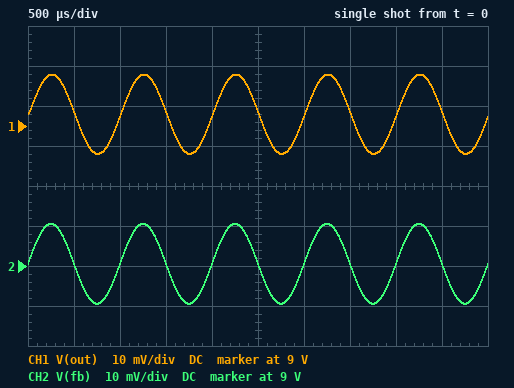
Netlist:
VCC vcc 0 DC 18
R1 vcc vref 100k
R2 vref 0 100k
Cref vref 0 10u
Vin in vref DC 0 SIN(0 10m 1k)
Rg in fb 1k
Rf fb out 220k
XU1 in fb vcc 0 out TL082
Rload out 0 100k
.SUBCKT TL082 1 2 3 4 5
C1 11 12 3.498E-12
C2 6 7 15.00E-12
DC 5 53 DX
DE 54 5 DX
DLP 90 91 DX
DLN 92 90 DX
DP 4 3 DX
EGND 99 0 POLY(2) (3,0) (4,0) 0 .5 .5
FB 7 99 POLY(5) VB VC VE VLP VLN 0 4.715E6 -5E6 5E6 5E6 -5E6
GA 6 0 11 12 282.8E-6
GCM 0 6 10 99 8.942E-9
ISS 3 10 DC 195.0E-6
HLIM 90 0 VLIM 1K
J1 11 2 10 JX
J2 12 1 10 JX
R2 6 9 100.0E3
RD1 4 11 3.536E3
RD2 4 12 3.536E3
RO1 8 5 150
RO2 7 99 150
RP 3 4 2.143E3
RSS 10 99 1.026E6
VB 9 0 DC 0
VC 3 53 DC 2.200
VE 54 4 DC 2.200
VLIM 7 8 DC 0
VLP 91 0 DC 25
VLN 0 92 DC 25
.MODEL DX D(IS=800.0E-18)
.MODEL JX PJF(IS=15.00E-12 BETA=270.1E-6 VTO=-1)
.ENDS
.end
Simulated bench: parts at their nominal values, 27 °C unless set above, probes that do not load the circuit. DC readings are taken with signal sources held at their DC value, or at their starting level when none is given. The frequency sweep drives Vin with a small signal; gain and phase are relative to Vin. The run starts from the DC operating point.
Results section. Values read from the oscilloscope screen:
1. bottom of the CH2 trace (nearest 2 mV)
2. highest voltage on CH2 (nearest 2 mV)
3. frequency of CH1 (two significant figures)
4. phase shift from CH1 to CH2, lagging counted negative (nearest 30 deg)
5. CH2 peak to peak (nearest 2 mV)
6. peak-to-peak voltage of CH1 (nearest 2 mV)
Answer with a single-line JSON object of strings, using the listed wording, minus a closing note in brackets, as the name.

{"bottom of the CH2 trace": "8.990 V", "highest voltage on CH2": "9.010 V", "frequency of CH1": "1.0 kHz", "phase shift from CH1 to CH2, lagging counted negative": "0 deg", "CH2 peak to peak": "20 mV", "peak-to-peak voltage of CH1": "20 mV"}
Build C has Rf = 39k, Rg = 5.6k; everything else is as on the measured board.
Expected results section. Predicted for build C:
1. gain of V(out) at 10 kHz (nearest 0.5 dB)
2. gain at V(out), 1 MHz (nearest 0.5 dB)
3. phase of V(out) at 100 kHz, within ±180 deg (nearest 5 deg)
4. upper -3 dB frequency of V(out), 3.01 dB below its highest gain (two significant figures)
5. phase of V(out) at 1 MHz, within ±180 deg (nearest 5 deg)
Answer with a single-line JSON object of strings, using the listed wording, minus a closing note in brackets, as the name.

{"gain of V(out) at 10 kHz": "0 dB", "gain at V(out), 1 MHz": "-7.5 dB", "phase of V(out) at 100 kHz, within ±180 deg": "-15 deg", "upper -3 dB frequency of V(out), 3.01 dB below its highest gain": "460 kHz", "phase of V(out) at 1 MHz, within ±180 deg": "-75 deg"}
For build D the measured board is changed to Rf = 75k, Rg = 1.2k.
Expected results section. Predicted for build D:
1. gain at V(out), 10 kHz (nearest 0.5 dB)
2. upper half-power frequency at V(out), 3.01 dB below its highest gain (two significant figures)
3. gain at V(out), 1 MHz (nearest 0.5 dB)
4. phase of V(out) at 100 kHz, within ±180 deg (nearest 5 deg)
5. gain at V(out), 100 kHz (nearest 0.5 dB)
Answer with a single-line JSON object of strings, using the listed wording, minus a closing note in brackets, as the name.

{"gain at V(out), 10 kHz": "0 dB", "upper half-power frequency at V(out), 3.01 dB below its highest gain": "55 kHz", "gain at V(out), 1 MHz": "-25.5 dB", "phase of V(out) at 100 kHz, within ±180 deg": "-60 deg", "gain at V(out), 100 kHz": "-6.5 dB"}
